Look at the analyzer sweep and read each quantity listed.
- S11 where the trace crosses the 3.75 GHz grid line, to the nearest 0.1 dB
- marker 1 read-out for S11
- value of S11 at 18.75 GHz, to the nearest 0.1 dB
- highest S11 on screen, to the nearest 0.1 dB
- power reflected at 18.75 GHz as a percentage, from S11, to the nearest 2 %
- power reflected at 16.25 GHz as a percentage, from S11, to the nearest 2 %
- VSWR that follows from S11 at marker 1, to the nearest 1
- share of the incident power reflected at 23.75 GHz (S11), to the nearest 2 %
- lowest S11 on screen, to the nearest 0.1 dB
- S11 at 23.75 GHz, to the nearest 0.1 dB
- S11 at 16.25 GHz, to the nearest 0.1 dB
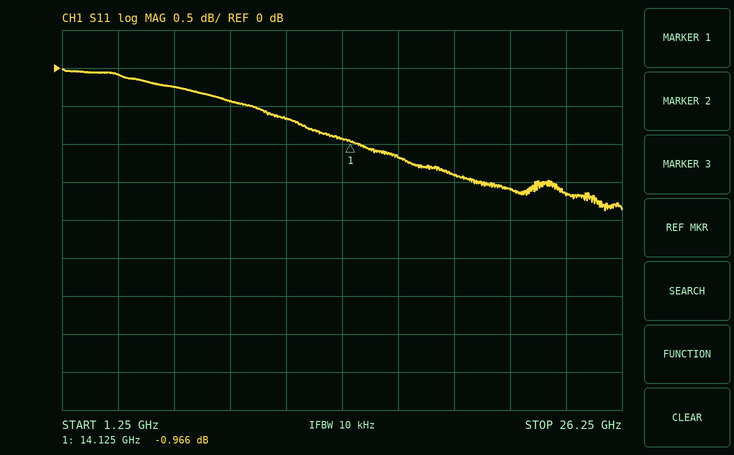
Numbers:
-0.1 dB
-0.966 dB
-1.4 dB
0.0 dB
72 %
76 %
18
68 %
-1.9 dB
-1.7 dB
-1.2 dB
